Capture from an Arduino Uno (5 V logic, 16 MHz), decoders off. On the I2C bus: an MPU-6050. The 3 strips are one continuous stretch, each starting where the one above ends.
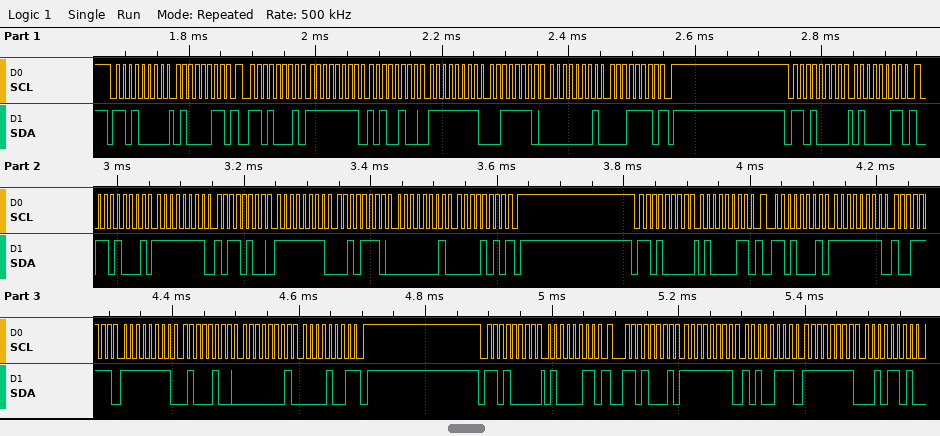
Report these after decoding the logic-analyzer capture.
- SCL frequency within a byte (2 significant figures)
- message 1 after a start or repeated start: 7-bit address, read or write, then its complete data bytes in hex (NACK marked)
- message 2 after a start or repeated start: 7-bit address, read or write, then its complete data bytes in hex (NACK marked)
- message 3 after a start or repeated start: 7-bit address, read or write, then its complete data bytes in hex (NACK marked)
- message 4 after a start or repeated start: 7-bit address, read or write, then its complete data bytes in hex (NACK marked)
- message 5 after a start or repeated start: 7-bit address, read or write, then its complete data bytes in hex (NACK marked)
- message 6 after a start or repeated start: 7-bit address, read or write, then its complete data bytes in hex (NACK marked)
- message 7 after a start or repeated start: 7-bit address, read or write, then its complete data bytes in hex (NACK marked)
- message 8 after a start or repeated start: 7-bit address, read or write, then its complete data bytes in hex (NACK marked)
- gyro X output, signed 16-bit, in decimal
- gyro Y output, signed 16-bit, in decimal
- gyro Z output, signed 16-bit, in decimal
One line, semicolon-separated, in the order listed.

100 kHz; 0x68 write: 43; 0x68 read: FF A4 FF 3E 01 1E NACK; 0x68 write: 43; 0x68 read: FF B4 FF 2E 01 0A NACK; 0x68 write: 43; 0x68 read: FF 9F FF 44 01 09 NACK; 0x68 write: 43; 0x68 read: FF A7 FF 2D; -92; -194; 286
